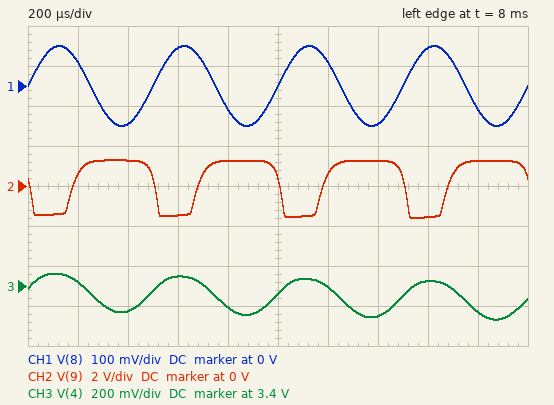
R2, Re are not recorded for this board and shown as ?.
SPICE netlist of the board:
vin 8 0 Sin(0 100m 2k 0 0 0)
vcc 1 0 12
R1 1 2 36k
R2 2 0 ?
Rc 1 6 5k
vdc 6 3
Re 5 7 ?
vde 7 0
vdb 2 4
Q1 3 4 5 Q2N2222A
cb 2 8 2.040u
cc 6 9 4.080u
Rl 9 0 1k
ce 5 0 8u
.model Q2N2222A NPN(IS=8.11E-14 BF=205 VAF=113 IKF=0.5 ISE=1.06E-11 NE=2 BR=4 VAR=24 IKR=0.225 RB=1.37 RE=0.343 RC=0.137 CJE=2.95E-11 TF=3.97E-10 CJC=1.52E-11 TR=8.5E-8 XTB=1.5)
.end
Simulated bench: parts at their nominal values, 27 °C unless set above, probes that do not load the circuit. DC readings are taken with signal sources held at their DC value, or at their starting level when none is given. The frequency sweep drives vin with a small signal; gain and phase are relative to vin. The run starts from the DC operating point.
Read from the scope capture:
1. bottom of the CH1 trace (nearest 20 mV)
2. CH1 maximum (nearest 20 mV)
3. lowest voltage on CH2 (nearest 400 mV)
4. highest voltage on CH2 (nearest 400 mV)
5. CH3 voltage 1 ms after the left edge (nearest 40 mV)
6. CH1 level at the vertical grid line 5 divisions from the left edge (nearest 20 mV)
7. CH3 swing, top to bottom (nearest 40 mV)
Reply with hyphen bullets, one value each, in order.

- -100 mV
- 100 mV
- -1.6 V
- 1.2 V
- 3.36 V
- 0 V
- 240 mV
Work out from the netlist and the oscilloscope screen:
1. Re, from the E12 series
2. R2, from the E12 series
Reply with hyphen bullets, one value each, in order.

- 1.8 kΩ
- 22 kΩ
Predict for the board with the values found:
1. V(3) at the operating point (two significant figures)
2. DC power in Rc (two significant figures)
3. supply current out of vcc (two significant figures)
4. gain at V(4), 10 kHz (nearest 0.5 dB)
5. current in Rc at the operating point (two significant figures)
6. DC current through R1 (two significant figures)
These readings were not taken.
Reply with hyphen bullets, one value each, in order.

- 3.3 V
- 15 mW
- 2.0 mA
- 0 dB
- 1.7 mA
- 230 µA
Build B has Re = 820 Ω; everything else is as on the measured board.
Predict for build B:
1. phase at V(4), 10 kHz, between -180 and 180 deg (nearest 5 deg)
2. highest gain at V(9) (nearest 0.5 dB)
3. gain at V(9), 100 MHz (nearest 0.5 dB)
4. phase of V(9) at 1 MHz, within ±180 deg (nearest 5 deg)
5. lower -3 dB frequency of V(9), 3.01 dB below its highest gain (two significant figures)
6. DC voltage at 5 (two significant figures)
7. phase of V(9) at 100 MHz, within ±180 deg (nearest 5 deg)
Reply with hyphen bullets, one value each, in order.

- 10 deg
- 8.5 dB
- -1.0 dB
- 145 deg
- 2.1 kHz
- 1.8 V
- 0 deg
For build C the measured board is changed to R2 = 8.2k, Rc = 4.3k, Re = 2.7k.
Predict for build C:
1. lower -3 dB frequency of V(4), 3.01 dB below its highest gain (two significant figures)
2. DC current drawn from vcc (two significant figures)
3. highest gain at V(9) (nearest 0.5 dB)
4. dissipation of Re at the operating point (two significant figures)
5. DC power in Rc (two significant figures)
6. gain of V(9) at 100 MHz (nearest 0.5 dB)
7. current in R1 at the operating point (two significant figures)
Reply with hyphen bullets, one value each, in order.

- 12 Hz
- 870 µA
- 25.5 dB
- 970 µW
- 1.5 mW
- 14.0 dB
- 270 µA
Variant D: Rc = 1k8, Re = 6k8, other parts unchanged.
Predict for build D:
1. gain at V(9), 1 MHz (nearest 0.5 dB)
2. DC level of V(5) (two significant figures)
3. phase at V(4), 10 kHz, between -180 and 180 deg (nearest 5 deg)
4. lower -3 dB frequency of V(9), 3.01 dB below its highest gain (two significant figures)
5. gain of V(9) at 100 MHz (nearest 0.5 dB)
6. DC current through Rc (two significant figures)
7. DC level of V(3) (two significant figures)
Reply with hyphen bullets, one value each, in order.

- 23.0 dB
- 3.9 V
- 0 deg
- 450 Hz
- 13.0 dB
- 570 µA
- 11 V
